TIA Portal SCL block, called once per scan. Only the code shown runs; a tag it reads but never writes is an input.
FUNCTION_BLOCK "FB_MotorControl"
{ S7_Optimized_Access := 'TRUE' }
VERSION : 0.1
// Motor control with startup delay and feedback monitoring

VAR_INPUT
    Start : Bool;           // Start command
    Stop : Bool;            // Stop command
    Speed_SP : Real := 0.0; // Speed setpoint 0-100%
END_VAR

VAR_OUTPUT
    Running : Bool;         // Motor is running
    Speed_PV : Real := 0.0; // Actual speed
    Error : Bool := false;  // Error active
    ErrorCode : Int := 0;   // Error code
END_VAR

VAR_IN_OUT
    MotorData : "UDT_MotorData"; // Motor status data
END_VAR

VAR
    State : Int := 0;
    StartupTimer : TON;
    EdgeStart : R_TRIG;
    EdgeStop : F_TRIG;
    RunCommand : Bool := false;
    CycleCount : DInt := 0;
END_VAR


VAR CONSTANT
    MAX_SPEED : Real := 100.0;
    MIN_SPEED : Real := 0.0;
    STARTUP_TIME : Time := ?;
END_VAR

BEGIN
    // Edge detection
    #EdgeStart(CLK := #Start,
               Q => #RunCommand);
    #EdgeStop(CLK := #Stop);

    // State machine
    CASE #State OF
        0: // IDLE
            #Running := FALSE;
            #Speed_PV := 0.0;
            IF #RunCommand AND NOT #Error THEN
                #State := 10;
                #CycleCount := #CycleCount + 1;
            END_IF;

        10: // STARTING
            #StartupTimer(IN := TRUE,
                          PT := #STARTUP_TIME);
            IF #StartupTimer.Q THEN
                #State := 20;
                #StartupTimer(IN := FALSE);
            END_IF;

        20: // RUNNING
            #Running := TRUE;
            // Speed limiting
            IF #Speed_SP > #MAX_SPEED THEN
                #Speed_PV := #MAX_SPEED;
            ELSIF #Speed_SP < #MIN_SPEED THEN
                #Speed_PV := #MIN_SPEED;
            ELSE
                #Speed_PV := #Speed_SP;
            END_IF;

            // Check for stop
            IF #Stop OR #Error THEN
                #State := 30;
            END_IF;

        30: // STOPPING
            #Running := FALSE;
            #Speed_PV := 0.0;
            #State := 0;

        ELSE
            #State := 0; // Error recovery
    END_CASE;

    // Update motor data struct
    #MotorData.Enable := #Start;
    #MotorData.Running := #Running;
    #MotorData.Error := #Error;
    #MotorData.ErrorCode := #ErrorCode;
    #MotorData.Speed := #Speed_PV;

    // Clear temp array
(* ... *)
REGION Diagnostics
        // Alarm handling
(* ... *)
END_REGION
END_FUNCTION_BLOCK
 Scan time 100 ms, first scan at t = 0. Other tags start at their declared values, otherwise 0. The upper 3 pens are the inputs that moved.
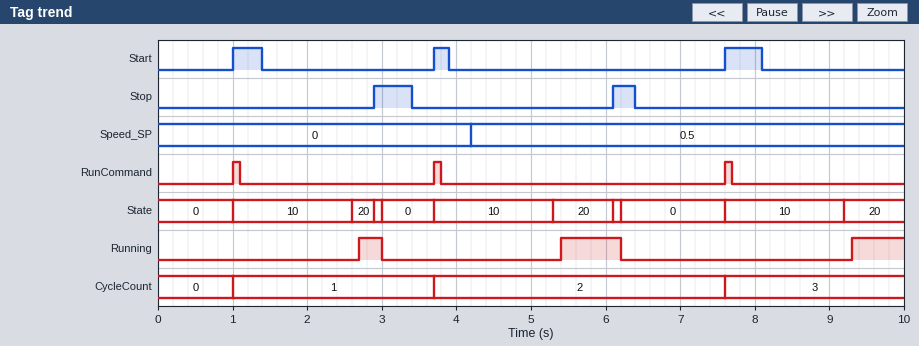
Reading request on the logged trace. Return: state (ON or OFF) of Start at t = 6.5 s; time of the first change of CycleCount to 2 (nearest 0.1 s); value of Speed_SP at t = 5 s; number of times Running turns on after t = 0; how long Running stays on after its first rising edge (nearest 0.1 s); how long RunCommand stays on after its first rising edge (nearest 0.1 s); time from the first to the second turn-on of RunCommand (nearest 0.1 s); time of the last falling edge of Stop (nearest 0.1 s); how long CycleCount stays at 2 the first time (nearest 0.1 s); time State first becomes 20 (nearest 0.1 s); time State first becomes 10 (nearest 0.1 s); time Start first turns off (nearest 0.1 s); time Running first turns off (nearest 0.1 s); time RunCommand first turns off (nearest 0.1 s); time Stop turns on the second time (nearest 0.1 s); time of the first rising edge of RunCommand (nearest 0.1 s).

OFF
3.7 s
0.5
3
0.3 s
0.1 s
2.7 s
6.4 s
3.9 s
2.6 s
1.0 s
1.4 s
3.0 s
1.1 s
6.1 s
1.0 s
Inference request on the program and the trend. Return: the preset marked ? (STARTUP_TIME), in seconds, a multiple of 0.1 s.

1.5 s
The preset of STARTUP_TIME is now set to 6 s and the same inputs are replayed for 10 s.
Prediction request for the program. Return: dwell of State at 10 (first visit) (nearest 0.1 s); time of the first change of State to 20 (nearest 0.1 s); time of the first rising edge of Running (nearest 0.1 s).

6.1 s
7.1 s
7.2 s
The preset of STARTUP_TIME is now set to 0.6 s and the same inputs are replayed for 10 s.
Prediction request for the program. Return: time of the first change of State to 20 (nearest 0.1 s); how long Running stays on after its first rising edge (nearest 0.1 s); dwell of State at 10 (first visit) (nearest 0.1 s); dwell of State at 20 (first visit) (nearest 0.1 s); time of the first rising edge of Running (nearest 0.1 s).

1.7 s
1.2 s
0.7 s
1.2 s
1.8 s
